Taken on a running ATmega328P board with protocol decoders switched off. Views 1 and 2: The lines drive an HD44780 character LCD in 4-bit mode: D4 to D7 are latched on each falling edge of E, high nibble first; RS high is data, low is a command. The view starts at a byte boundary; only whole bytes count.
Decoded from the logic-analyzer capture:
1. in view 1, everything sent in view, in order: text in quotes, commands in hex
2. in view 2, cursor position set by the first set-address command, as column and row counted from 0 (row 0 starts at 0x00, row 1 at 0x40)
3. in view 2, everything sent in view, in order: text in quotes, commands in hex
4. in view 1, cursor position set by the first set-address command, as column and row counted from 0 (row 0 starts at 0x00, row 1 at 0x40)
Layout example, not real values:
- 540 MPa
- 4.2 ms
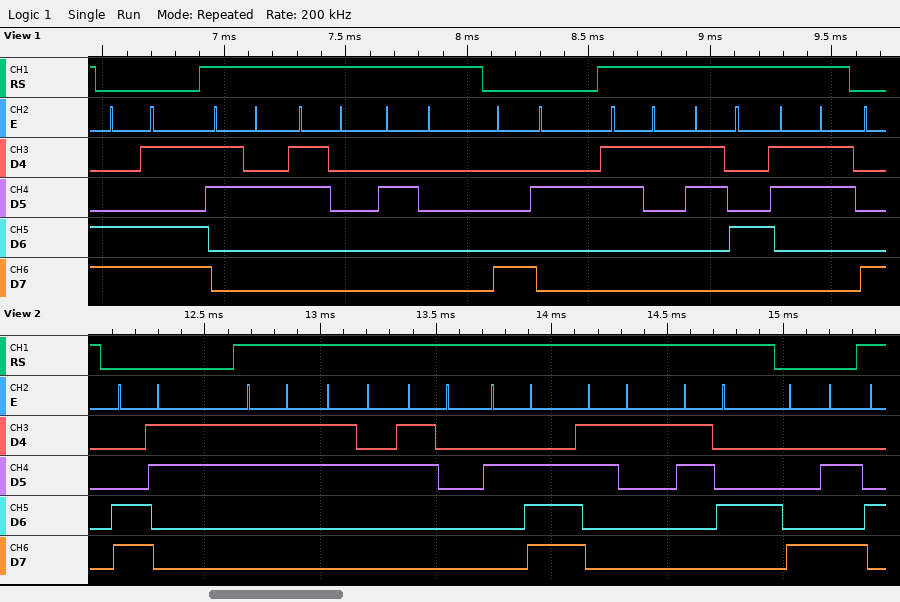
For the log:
- 0xCD "20 " 0x82 "143"
- column 3, row 1
- 0xC3 "320.14" 0x8A
- column 13, row 1
